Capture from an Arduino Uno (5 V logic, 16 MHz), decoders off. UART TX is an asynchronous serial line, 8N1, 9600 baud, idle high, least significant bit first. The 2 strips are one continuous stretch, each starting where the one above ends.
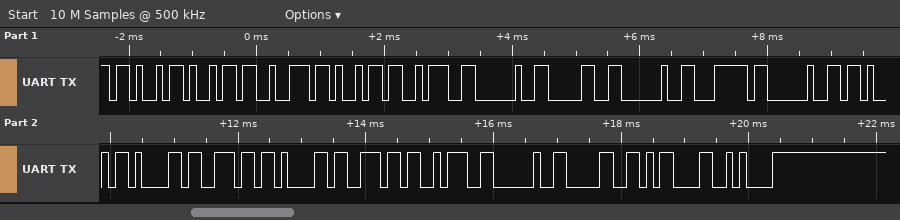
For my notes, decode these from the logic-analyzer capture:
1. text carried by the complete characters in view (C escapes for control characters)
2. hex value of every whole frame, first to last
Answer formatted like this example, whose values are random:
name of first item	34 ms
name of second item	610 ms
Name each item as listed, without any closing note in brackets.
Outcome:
text carried by the complete characters in view	"Kiri: 0 | Kanan: 0\r\n"
hex value of every whole frame, first to last	4B 69 72 69 3A 20 30 20 7C 20 4B 61 6E 61 6E 3A 20 30 0D 0A
